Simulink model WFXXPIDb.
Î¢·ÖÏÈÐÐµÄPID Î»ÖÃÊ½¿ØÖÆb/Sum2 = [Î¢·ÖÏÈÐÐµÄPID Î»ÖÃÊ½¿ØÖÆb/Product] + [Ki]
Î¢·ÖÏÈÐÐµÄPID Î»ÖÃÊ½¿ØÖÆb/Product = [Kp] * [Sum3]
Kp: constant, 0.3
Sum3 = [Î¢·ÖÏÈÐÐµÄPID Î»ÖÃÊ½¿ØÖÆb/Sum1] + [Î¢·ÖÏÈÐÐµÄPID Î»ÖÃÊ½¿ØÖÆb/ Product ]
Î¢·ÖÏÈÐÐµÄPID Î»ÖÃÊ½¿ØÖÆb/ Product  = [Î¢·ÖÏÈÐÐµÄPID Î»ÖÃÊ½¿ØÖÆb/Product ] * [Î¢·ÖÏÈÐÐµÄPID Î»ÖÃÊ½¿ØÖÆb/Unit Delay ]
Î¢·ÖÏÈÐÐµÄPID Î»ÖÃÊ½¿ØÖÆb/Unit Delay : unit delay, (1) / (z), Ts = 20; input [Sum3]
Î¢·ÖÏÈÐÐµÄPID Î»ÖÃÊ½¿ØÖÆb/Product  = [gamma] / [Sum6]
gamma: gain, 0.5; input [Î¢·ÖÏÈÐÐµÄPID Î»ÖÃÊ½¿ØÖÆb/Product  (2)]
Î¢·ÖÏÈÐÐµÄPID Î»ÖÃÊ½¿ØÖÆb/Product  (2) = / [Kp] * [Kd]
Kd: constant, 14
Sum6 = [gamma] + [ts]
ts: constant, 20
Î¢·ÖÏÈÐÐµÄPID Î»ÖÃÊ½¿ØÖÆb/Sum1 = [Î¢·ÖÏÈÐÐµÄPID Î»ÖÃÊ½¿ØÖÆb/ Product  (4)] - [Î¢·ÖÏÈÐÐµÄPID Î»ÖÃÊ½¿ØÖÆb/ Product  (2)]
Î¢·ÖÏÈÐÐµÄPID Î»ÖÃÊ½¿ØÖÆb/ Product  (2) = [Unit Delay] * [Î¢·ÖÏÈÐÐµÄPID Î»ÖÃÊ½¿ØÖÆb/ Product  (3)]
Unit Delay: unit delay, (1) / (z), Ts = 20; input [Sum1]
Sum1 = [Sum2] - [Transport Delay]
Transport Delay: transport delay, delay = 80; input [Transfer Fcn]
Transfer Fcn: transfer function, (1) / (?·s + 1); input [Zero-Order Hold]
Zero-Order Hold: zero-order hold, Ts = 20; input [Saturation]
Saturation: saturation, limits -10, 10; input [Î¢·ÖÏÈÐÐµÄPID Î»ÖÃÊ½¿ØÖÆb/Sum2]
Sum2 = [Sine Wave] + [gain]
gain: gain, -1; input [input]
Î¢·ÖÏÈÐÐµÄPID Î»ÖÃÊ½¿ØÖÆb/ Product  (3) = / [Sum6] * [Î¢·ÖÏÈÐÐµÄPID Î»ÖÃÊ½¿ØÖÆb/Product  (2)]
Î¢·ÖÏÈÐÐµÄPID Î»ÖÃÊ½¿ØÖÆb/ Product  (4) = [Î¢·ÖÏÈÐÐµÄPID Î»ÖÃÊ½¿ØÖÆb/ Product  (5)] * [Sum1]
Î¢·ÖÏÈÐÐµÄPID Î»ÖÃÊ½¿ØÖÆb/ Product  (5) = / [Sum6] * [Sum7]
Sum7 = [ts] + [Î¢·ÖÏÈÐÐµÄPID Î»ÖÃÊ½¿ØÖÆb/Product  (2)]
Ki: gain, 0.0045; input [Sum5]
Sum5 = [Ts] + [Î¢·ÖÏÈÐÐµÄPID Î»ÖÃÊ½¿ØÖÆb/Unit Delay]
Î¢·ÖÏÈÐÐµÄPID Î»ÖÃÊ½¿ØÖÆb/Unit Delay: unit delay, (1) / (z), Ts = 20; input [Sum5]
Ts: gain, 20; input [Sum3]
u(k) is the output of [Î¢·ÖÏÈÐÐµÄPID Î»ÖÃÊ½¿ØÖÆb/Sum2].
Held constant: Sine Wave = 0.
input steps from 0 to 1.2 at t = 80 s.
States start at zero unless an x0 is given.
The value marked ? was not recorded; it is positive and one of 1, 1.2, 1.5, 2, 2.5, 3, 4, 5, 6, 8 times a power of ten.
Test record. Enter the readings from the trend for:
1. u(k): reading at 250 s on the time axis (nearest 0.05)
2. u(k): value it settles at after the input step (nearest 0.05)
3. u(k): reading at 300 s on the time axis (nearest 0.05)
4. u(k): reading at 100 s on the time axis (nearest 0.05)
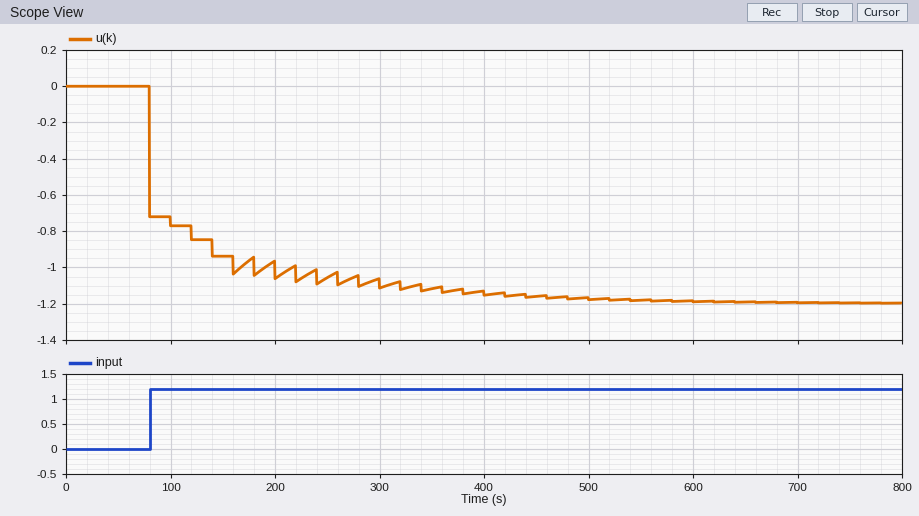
-1.05
-1.20
-1.10
-0.75
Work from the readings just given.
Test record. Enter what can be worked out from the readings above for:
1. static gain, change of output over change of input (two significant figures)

-1.0
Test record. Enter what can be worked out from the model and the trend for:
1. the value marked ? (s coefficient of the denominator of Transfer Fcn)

80
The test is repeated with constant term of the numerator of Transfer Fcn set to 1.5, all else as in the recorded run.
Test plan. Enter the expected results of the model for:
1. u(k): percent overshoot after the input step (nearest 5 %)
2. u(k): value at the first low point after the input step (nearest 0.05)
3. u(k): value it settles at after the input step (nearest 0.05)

30 %
-1.05
-0.80
